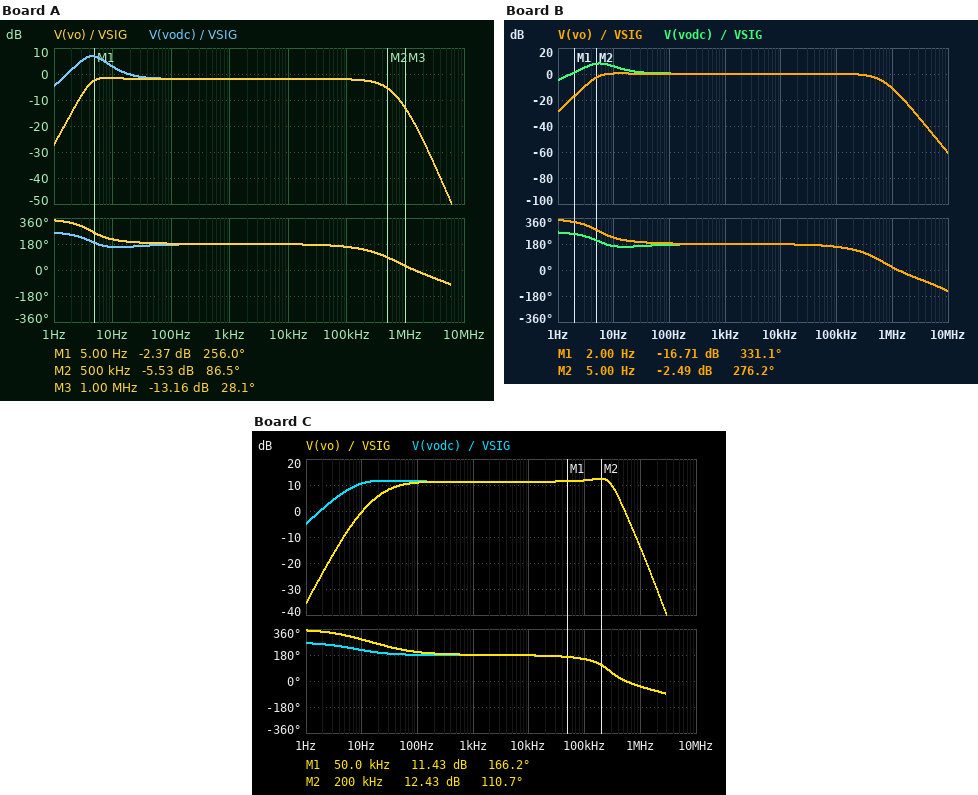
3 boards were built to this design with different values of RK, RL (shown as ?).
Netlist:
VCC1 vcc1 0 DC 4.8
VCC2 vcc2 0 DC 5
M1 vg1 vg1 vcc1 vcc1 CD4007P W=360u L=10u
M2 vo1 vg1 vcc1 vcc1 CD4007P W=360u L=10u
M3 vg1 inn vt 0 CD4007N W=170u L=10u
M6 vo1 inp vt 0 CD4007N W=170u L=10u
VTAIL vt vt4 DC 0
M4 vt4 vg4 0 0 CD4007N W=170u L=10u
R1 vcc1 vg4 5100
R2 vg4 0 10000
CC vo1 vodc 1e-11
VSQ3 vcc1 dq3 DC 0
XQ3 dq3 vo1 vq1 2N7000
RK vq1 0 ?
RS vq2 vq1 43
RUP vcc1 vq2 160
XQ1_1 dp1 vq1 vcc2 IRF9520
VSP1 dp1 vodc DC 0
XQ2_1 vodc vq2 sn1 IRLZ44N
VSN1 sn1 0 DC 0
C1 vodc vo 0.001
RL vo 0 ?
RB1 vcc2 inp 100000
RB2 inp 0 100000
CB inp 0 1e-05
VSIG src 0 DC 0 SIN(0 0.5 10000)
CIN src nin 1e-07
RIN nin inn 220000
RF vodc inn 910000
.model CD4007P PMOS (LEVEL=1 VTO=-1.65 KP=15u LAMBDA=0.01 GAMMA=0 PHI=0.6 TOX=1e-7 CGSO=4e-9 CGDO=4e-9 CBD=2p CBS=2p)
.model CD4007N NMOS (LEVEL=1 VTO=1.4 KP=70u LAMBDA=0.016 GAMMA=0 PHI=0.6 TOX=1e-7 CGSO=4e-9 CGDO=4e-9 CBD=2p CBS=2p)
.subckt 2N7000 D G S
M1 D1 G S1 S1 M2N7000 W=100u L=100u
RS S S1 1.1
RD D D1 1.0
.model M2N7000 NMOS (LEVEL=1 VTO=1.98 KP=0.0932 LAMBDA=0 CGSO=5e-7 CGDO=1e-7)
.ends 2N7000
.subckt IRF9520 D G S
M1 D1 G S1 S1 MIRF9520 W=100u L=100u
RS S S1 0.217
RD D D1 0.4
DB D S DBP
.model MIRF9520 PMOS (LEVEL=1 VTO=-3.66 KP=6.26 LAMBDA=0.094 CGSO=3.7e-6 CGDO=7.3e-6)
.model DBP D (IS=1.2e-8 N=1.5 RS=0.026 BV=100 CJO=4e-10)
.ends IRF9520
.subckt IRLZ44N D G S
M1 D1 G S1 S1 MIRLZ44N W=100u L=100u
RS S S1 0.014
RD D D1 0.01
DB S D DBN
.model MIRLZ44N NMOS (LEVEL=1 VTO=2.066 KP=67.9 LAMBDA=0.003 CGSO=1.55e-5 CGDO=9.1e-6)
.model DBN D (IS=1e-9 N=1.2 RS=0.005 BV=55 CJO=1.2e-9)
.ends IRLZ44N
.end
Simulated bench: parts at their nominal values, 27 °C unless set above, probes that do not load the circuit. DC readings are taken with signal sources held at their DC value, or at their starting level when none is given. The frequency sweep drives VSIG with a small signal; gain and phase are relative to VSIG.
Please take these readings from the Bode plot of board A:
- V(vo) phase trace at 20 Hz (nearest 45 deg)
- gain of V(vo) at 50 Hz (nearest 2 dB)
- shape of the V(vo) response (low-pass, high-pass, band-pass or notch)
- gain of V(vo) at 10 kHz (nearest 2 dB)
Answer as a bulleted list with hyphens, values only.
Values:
- 180 deg
- -2 dB
- band-pass
- -2 dB
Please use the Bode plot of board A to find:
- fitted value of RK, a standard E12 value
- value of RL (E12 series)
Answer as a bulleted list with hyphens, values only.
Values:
- 22 Ω
- 12 Ω
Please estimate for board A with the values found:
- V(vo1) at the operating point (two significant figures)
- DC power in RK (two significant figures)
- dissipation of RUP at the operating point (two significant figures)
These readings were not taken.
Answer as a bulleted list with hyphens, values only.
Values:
- 4.3 V
- 81 mW
- 47 mW
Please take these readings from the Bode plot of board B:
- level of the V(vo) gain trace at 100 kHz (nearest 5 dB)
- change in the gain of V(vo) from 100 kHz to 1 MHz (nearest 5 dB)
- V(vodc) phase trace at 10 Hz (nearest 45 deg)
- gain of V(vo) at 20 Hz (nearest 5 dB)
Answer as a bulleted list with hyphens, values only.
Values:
- 0 dB
- -10 dB
- 180 deg
- 0 dB
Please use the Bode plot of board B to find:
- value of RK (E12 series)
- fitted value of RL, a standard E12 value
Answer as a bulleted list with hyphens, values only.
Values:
- 27 Ω
- 10 Ω
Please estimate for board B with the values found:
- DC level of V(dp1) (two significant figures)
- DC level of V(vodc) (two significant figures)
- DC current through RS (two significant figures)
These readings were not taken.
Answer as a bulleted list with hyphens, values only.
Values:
- 2.6 V
- 2.6 V
- 17 mA
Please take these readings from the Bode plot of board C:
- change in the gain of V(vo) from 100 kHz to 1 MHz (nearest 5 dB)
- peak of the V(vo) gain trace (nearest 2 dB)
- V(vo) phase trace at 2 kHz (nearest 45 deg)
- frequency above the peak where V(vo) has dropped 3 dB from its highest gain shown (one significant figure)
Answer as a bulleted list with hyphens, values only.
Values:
- -25 dB
- 12 dB
- 180 deg
- 300 kHz
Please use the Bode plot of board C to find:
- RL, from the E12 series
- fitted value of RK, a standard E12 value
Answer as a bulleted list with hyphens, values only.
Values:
- 4.7 Ω
- 68 Ω
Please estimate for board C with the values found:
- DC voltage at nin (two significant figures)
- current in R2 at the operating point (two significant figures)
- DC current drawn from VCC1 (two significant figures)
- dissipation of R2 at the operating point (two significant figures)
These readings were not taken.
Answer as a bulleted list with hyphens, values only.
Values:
- 2.5 V
- 320 µA
- 21 mA
- 1.0 mW
